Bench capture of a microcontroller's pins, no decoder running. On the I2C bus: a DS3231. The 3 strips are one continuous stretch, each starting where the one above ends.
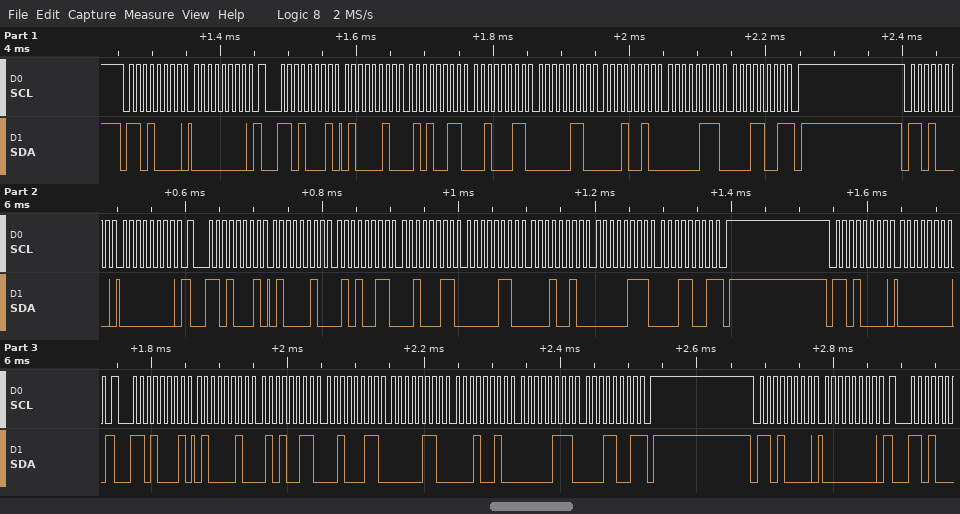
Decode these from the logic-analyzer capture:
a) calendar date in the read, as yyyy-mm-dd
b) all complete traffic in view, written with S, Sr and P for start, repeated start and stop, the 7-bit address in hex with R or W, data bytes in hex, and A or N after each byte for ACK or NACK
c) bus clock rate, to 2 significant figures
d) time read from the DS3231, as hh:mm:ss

2019-07-12
S 68W A 00 A Sr 68R A 42 A 53 A 23 A 06 A 12 A 07 A 19 N P S 68W A 00 A Sr 68R A 42 A 53 A 23 A 06 A 12 A 07 A 19 N P S 68W A 00 A Sr 68R A 42 A 53 A 23 A 06 A 12 A 07 A 19 N P S 68W A 00 A
100 kHz
23:53:42
